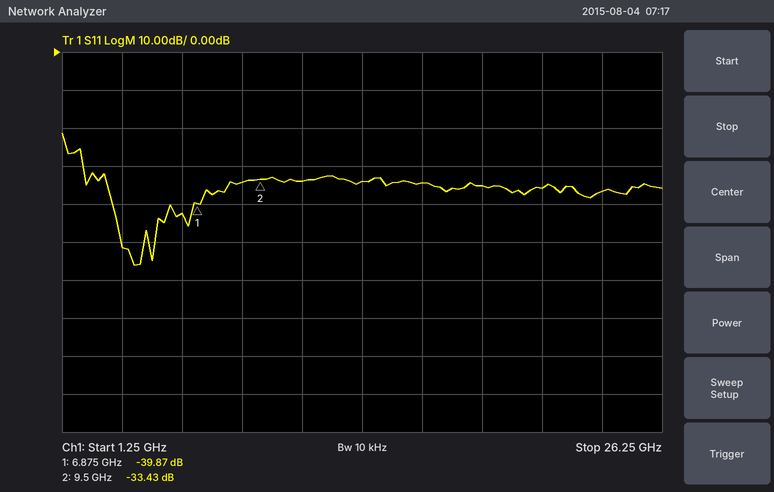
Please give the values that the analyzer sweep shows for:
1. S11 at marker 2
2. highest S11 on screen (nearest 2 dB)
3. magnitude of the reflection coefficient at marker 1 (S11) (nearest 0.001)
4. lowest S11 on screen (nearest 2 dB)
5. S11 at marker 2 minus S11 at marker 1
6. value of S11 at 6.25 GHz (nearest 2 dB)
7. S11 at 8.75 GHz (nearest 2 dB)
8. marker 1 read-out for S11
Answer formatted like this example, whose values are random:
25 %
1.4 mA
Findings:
-33.43 dB
-22 dB
0.010
-56 dB
6.44 dB
-42 dB
-34 dB
-39.87 dB
